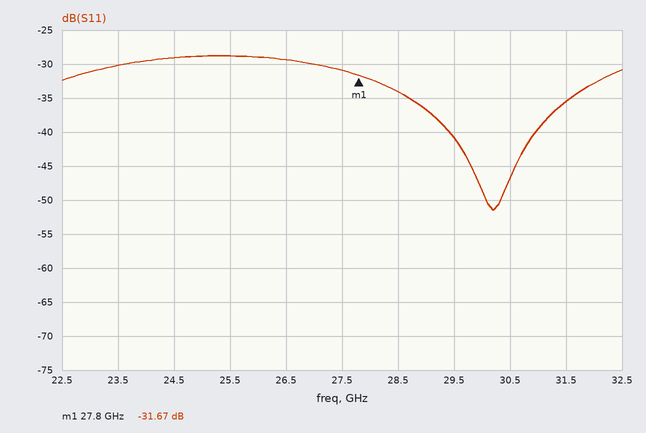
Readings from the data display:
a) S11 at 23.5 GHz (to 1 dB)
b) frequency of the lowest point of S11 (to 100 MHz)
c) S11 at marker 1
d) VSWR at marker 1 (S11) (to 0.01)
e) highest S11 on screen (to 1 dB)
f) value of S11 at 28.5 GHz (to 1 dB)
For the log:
-30 dB
30.2 GHz
-31.67 dB
1.05
-29 dB
-34 dB
